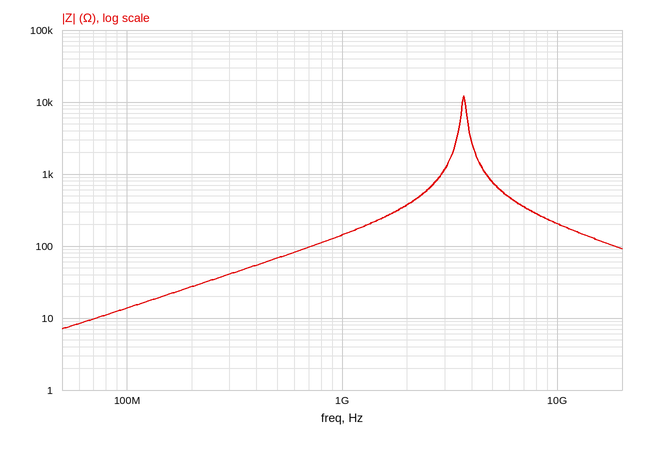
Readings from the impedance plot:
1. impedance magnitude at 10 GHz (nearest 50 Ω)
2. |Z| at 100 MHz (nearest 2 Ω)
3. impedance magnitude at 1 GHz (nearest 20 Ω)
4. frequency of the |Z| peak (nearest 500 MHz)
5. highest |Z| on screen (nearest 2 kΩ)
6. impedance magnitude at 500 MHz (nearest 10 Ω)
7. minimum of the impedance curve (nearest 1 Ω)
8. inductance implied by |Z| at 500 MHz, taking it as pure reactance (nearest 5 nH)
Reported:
200 Ω
14 Ω
140 Ω
3.5 GHz
12 kΩ
70 Ω
7 Ω
20 nH
